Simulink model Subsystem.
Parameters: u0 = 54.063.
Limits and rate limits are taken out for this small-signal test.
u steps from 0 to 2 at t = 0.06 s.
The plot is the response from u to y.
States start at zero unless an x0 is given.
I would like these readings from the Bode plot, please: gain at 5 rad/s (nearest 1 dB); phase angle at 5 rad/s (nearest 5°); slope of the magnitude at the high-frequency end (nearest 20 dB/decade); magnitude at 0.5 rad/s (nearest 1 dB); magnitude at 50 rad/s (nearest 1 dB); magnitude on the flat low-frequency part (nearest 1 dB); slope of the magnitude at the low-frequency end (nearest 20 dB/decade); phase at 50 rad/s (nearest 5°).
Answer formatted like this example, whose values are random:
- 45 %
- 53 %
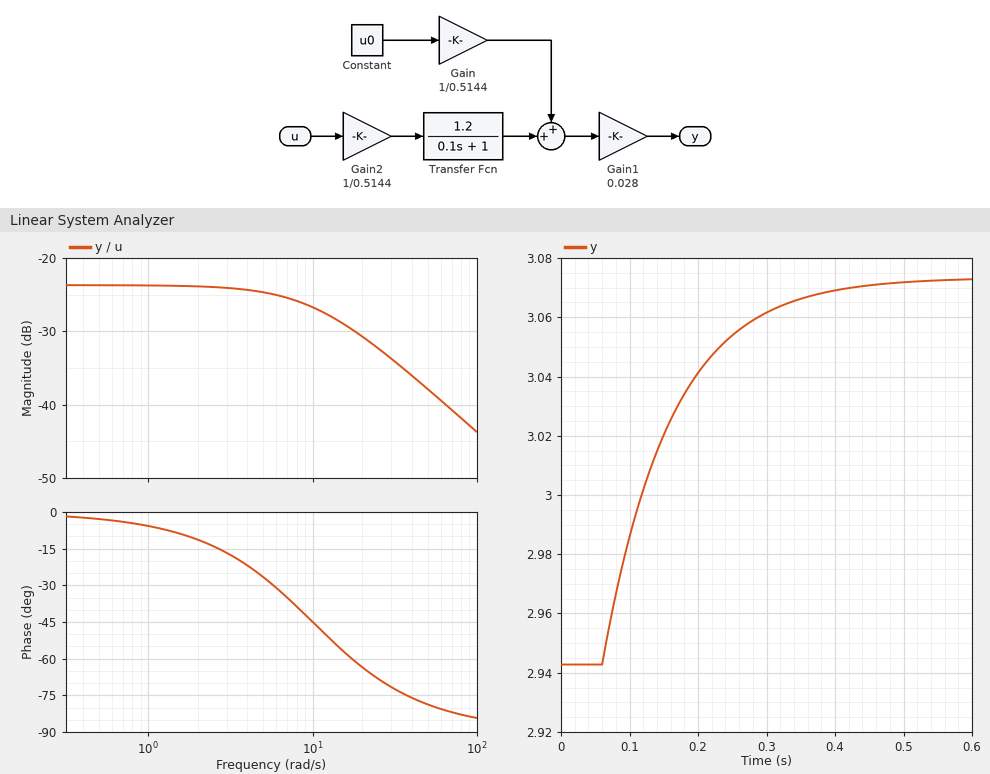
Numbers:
- -25 dB
- -25°
- -20 dB/decade
- -24 dB
- -38 dB
- -24 dB
- 0 dB/decade
- -80°
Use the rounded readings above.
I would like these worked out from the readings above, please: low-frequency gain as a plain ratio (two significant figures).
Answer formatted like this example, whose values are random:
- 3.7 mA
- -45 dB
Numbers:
- 0.063
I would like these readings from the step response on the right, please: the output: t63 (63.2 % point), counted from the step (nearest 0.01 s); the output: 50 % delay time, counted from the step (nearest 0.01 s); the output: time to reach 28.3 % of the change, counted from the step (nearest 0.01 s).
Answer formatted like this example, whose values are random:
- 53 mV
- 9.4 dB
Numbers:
- 0.10 s
- 0.07 s
- 0.03 s
